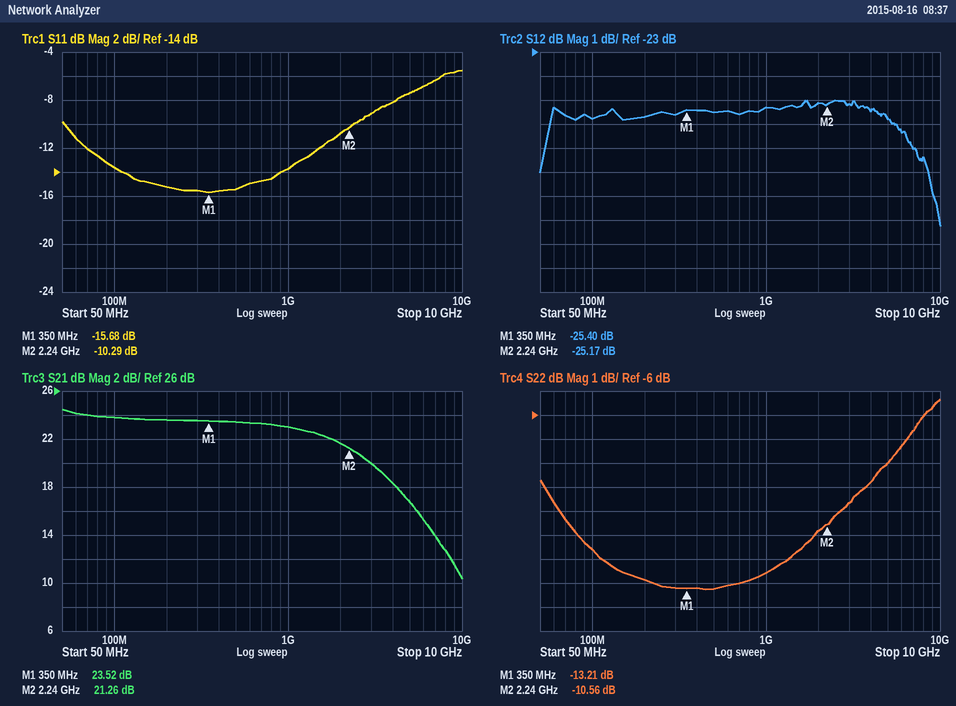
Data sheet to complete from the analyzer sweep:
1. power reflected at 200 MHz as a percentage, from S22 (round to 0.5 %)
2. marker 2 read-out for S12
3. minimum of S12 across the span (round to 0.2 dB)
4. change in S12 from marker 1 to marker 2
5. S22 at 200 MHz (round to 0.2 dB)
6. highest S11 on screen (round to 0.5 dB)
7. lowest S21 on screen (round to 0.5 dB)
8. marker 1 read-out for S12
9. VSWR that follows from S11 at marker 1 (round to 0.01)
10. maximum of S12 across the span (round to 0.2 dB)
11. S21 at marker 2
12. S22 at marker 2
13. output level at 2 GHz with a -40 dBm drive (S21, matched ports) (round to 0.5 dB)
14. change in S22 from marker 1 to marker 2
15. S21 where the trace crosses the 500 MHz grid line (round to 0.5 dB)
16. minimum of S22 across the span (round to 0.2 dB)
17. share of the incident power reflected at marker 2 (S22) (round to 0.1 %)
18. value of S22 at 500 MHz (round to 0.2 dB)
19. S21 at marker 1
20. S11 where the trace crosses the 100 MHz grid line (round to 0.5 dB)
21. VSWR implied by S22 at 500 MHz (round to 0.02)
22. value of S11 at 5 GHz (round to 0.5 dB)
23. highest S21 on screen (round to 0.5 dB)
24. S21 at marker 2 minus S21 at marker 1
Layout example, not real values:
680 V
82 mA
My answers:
5.0 %
-25.17 dB
-30.2 dB
0.23 dB
-12.8 dB
-5.5 dB
10.5 dB
-25.40 dB
1.39
-25.0 dB
21.26 dB
-10.56 dB
-18.5 dBm
2.65 dB
23.5 dB
-13.2 dB
8.8 %
-13.2 dB
23.52 dB
-13.5 dB
1.56
-7.5 dB
24.5 dB
-2.26 dB
